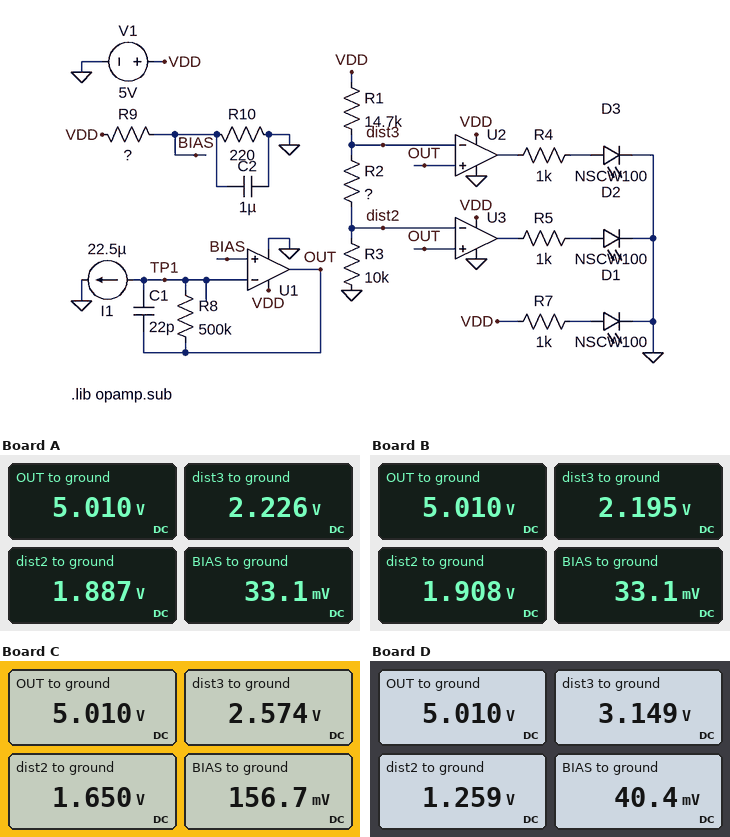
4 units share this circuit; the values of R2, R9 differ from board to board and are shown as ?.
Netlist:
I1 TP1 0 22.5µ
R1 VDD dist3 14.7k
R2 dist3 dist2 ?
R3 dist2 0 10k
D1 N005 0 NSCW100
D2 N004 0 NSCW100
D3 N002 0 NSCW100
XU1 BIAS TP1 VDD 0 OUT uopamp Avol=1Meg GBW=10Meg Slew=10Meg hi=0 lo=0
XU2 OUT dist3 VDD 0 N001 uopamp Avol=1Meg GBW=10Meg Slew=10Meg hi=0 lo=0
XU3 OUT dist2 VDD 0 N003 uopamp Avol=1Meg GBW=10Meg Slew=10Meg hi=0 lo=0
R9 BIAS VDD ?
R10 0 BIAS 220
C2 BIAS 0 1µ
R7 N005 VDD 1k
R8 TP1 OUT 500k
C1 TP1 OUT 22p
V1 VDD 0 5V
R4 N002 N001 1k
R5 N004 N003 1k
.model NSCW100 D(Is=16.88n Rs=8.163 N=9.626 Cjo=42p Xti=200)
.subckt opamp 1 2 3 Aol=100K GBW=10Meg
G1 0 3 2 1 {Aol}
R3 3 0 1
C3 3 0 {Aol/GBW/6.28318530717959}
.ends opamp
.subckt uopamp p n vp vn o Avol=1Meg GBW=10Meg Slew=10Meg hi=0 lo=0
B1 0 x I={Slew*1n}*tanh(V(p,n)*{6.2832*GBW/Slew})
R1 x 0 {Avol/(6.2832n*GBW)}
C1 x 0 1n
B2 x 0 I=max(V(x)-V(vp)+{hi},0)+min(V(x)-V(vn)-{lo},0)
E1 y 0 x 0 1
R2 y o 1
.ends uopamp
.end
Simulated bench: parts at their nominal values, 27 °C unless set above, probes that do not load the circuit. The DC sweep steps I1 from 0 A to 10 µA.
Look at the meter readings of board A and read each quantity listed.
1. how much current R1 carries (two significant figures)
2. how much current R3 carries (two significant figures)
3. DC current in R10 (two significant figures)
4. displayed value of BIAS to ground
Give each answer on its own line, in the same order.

190 µA
190 µA
150 µA
33.1 mV
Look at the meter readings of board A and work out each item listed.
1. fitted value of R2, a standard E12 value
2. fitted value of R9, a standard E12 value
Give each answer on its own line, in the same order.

1.8 kΩ
33 kΩ
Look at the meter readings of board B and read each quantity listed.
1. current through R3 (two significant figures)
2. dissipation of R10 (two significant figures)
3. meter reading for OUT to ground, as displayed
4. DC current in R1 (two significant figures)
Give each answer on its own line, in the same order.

190 µA
5.0 µW
5.010 V
190 µA
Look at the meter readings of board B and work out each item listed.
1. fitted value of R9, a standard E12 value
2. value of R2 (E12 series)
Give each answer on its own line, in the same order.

33 kΩ
1.5 kΩ
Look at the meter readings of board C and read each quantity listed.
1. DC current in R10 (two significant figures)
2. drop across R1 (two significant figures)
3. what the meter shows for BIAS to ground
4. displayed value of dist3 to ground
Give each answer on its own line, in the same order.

710 µA
2.4 V
156.7 mV
2.574 V
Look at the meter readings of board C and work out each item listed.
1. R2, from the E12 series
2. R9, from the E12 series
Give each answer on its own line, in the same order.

5.6 kΩ
6.8 kΩ
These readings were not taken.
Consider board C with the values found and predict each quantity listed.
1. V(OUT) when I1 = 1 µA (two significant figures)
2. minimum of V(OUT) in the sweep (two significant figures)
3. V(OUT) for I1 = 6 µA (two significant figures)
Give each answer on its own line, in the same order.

660 mV
160 mV
3.2 V
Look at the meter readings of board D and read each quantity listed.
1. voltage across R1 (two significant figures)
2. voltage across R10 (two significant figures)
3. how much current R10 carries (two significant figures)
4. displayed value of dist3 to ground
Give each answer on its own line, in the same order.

1.9 V
40 mV
180 µA
3.149 V
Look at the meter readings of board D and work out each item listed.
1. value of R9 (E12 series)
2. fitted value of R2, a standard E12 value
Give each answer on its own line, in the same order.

27 kΩ
15 kΩ
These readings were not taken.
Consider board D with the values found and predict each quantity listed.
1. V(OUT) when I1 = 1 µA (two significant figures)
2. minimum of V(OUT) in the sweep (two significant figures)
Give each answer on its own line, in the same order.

540 mV
40 mV
